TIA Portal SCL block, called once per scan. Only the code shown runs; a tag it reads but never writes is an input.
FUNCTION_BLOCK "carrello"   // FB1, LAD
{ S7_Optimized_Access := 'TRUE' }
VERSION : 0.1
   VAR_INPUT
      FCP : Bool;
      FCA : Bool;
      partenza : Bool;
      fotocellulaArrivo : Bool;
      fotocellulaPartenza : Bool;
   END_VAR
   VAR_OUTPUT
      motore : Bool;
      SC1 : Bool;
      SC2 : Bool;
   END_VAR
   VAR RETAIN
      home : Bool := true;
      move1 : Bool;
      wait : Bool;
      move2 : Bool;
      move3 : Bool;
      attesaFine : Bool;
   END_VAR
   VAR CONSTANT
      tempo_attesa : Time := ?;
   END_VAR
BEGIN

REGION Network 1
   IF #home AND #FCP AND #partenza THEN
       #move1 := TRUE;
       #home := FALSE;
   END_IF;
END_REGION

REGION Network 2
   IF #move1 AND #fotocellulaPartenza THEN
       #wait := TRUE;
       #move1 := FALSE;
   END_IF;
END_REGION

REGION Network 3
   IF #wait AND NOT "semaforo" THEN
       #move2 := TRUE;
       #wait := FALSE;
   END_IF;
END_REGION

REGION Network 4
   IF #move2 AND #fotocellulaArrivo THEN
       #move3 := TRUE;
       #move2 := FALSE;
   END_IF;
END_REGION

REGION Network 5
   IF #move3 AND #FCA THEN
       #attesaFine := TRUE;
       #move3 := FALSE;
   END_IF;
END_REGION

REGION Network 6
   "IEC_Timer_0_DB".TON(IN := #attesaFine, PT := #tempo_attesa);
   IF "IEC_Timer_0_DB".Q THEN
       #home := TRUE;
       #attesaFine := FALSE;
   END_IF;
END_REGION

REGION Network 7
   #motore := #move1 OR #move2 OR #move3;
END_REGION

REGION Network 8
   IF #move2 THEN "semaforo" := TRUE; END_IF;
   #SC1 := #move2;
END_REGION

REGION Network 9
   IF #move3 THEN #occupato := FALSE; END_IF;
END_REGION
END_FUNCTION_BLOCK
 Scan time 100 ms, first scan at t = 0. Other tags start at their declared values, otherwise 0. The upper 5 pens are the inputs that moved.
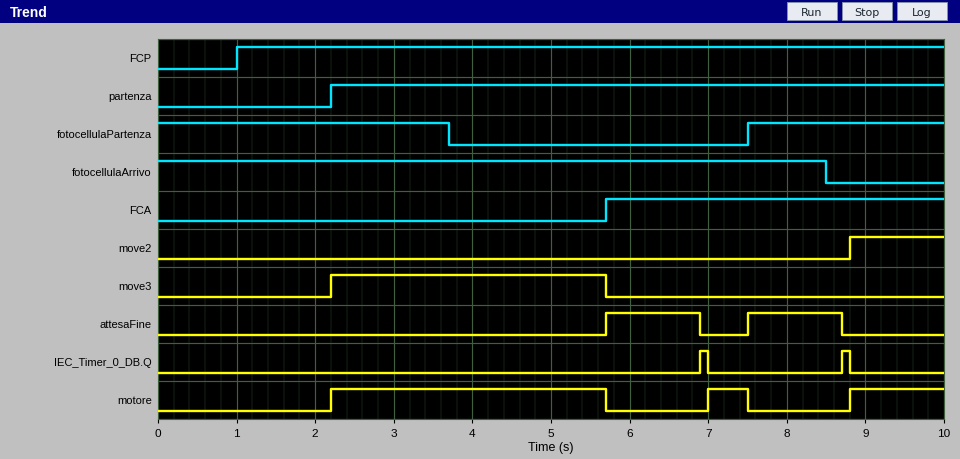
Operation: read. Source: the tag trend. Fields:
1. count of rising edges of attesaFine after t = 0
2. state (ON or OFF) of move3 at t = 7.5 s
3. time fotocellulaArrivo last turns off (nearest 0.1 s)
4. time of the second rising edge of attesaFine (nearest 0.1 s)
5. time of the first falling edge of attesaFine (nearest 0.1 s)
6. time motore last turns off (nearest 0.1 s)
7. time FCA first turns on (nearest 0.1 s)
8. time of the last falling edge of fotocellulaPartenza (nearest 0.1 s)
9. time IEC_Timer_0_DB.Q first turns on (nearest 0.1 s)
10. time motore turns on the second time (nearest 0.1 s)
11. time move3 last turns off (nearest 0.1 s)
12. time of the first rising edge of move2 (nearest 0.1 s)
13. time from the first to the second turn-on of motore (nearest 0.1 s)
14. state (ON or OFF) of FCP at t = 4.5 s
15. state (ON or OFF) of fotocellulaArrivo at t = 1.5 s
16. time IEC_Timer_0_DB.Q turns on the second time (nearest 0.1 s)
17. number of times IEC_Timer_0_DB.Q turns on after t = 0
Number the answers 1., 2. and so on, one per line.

1. 2
2. OFF
3. 8.5 s
4. 7.5 s
5. 6.9 s
6. 7.5 s
7. 5.7 s
8. 3.7 s
9. 6.9 s
10. 7.0 s
11. 5.7 s
12. 8.8 s
13. 4.8 s
14. ON
15. ON
16. 8.7 s
17. 2
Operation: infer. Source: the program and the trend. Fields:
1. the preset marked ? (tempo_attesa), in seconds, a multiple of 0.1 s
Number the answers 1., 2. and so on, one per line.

1. 1.2 s
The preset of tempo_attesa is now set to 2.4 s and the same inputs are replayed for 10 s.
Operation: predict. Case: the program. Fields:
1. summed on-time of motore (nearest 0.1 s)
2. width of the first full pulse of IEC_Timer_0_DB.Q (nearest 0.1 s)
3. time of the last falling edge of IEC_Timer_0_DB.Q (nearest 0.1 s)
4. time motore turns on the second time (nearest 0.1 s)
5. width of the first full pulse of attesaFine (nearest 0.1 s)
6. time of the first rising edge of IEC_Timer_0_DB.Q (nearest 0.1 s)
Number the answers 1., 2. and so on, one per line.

1. 5.0 s
2. 0.4 s
3. 8.5 s
4. 8.5 s
5. 2.4 s
6. 8.1 s
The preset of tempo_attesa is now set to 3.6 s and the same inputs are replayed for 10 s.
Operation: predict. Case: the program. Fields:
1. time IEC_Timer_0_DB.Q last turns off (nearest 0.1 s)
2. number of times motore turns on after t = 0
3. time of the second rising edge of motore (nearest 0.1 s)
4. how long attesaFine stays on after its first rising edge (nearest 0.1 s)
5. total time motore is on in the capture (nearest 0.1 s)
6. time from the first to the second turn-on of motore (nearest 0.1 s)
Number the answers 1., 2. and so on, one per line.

1. 9.4 s
2. 2
3. 9.4 s
4. 3.6 s
5. 4.1 s
6. 7.2 s
